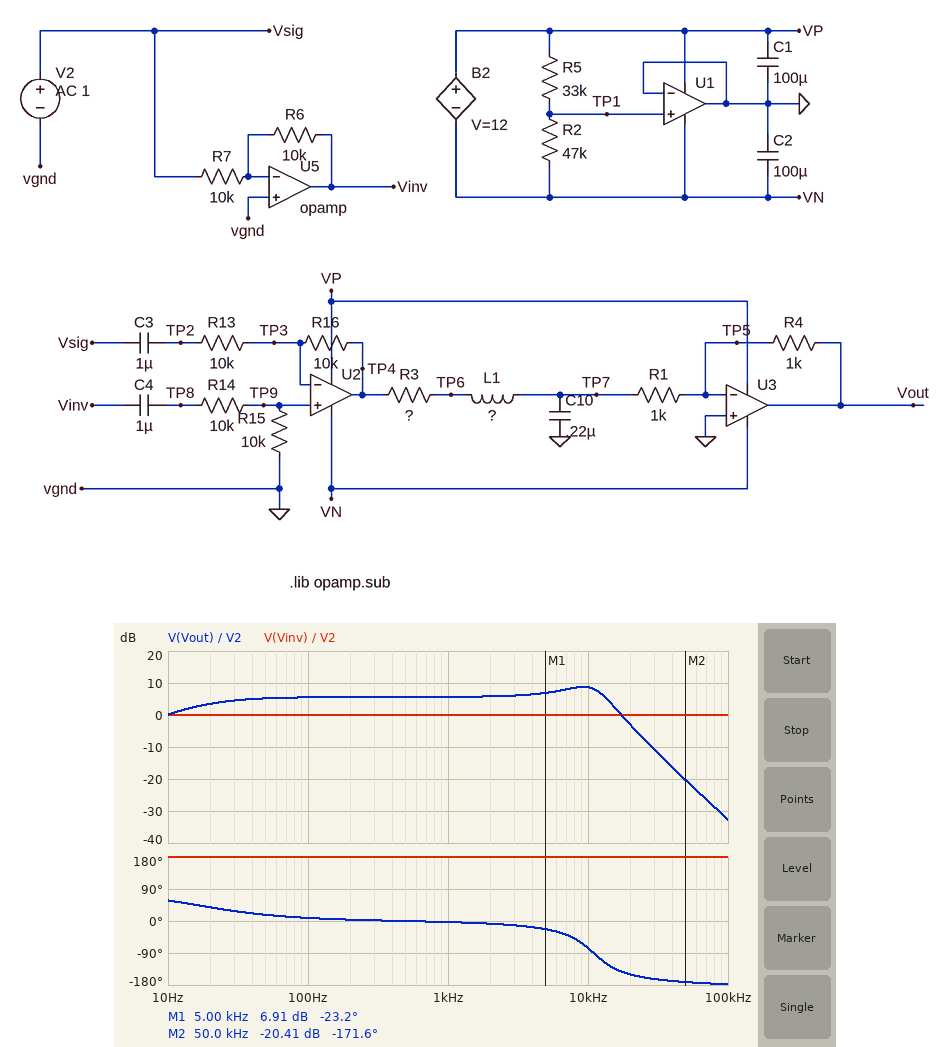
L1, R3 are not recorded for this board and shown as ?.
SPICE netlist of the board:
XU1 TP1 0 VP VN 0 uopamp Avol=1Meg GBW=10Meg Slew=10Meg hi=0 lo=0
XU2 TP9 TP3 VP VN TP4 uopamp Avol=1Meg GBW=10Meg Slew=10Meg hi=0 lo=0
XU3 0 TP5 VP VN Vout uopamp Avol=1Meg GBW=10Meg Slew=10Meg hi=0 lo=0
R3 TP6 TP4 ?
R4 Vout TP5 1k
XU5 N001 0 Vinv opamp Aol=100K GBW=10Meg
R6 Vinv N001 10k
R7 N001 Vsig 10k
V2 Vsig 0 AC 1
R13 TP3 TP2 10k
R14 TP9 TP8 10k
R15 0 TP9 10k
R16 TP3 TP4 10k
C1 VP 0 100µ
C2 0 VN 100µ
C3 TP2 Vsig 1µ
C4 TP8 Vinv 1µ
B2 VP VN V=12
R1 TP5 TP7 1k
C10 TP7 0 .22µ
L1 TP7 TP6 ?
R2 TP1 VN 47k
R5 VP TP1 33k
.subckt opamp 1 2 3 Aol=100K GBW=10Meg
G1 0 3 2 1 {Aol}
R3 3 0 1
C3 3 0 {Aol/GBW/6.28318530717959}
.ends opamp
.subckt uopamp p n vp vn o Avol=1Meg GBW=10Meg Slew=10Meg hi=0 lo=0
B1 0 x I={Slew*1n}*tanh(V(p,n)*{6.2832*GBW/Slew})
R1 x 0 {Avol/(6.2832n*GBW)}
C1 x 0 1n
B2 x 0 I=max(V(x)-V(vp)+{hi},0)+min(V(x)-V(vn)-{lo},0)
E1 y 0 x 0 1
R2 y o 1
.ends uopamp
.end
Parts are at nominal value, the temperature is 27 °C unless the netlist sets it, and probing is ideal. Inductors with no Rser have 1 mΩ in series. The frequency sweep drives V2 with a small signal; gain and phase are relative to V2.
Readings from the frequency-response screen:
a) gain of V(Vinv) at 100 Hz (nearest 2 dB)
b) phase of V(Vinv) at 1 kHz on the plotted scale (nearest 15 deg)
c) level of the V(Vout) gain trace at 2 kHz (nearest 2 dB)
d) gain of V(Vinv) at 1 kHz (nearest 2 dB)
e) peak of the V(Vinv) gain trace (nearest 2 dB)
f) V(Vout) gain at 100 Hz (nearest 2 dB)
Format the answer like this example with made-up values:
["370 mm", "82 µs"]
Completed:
["0 dB", "180 deg", "6 dB", "0 dB", "0 dB", "6 dB"]
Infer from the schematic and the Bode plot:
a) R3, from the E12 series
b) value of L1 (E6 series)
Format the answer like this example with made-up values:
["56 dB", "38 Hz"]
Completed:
["47 Ω", "1 mH"]
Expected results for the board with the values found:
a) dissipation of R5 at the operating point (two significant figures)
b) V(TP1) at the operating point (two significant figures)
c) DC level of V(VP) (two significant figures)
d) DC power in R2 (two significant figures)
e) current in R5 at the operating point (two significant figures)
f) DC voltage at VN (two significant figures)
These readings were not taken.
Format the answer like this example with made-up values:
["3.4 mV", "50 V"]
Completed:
["740 µW", "3.5 V", "8.5 V", "1.1 mW", "150 µA", "-3.5 V"]
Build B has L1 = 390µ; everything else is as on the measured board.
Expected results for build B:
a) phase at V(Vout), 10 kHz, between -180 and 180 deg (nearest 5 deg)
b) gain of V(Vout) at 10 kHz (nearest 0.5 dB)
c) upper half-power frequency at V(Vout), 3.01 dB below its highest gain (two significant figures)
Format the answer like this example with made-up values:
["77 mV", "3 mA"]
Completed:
["-45 deg", "6.0 dB", "20 kHz"]
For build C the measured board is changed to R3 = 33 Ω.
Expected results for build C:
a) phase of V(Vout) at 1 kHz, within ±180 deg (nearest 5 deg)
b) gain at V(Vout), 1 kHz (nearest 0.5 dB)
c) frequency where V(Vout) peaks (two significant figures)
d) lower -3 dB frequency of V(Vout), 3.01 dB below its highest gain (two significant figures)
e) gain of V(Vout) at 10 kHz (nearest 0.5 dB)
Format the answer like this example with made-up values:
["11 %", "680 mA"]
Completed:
["0 deg", "6.0 dB", "10 kHz", "6.2 kHz", "11.5 dB"]
